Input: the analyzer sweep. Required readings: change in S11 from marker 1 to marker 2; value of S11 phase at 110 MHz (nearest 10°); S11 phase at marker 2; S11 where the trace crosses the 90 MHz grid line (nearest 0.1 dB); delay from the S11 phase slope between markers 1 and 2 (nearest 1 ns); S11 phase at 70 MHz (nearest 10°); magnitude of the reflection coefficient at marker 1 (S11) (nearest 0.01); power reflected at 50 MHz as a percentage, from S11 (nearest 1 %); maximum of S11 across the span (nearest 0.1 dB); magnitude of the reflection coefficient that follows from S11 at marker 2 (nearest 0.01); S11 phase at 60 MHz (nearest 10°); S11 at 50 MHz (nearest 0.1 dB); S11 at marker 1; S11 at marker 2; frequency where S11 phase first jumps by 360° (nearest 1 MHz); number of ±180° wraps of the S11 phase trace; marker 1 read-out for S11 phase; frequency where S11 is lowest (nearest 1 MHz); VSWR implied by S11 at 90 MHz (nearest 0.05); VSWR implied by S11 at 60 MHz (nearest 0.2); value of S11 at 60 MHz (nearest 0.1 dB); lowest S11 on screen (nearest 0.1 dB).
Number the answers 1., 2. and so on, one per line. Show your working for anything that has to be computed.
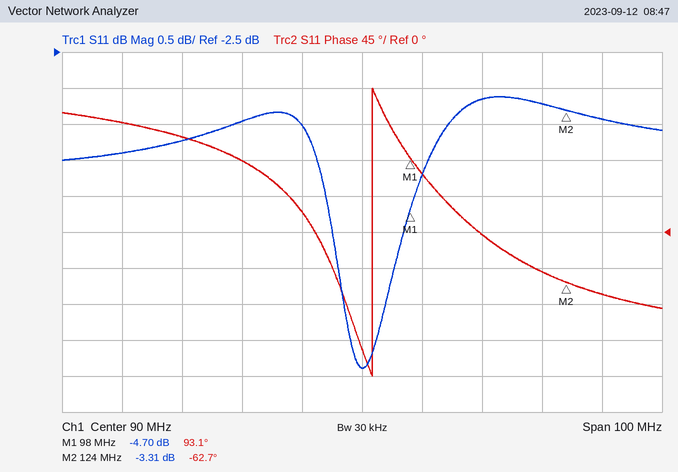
1. -3.31 − (-4.7) = 1.39 dB
2. 0°
3. -62.7°
4. -6.9 dB
5. −(-62.7° − (93.1°))/(360° × 26 MHz) ≈ 17 ns
6. 90°
7. 10^(-4.7/20) ≈ 0.58
8. 10^(-3.9/10) ≈ 41 %
9. -3.1 dB
10. 10^(-3.31/20) ≈ 0.68
11. 120°
12. -3.9 dB
13. -4.70 dB
14. -3.31 dB
15. 92 MHz
16. 1
17. 93.1°
18. 90 MHz
19. |Γ| = 10^(-6.9/20) = 0.4519; VSWR = (1 + 0.4519)/(1 − 0.4519) ≈ 2.65
20. |Γ| = 10^(-3.7/20) = 0.6531; VSWR = (1 + 0.6531)/(1 − 0.6531) ≈ 4.8
21. -3.7 dB
22. -6.9 dB
